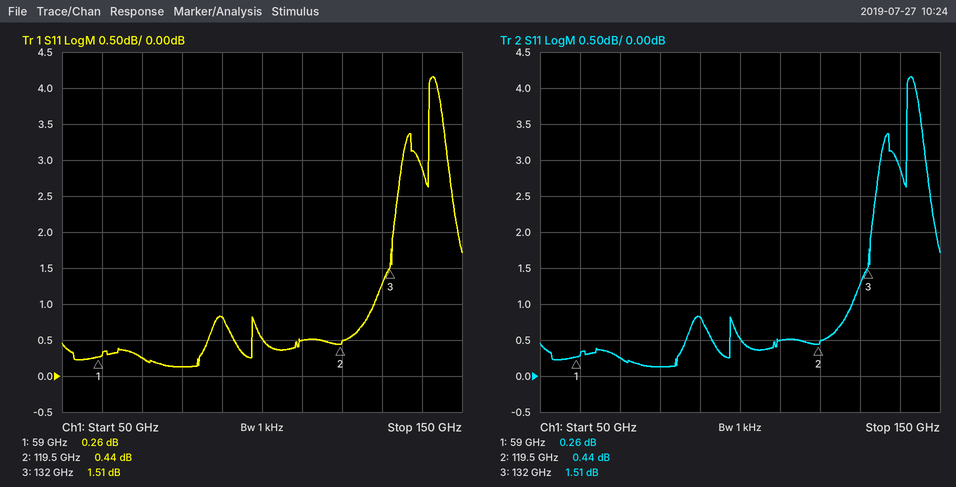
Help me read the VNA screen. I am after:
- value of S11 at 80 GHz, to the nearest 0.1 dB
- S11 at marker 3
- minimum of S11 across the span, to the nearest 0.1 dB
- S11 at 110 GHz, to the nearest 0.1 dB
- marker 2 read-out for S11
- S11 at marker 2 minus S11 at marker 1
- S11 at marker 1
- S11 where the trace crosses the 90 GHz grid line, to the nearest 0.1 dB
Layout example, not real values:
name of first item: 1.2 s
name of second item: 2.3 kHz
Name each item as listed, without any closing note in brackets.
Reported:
value of S11 at 80 GHz, to the nearest 0.1 dB: 0.1 dB
S11 at marker 3: 1.51 dB
minimum of S11 across the span, to the nearest 0.1 dB: 0.1 dB
S11 at 110 GHz, to the nearest 0.1 dB: 0.5 dB
marker 2 read-out for S11: 0.44 dB
S11 at marker 2 minus S11 at marker 1: 0.18 dB
S11 at marker 1: 0.26 dB
S11 where the trace crosses the 90 GHz grid line, to the nearest 0.1 dB: 0.8 dB
